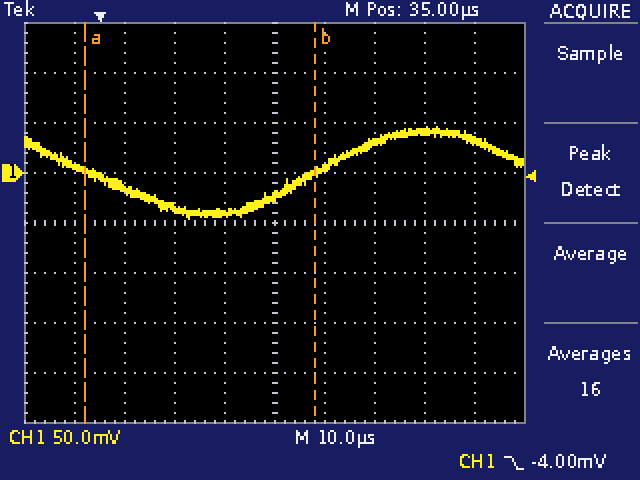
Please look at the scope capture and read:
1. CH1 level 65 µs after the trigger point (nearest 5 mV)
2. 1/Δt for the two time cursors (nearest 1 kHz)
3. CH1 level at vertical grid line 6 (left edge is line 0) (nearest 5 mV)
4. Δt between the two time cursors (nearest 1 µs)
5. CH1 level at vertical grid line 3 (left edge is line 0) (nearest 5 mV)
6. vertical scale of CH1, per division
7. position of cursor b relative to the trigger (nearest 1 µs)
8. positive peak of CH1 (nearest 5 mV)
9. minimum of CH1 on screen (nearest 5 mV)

40 mV
22 kHz
5 mV
46 µs
-35 mV
50 mV
+43 µs
45 mV
-45 mV
